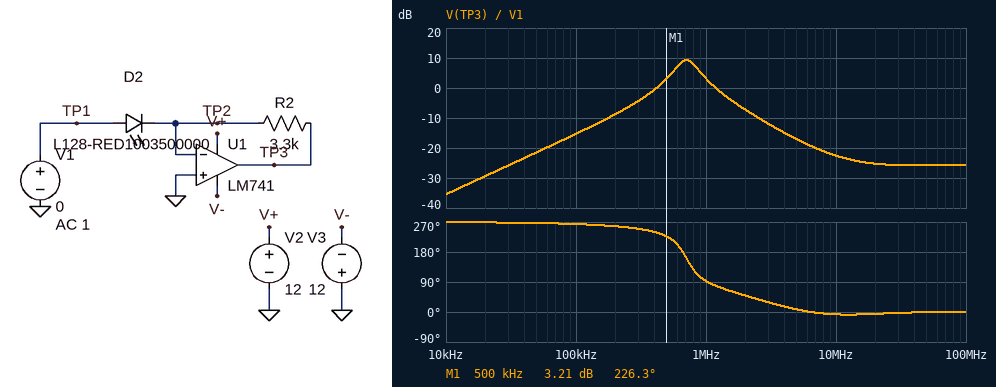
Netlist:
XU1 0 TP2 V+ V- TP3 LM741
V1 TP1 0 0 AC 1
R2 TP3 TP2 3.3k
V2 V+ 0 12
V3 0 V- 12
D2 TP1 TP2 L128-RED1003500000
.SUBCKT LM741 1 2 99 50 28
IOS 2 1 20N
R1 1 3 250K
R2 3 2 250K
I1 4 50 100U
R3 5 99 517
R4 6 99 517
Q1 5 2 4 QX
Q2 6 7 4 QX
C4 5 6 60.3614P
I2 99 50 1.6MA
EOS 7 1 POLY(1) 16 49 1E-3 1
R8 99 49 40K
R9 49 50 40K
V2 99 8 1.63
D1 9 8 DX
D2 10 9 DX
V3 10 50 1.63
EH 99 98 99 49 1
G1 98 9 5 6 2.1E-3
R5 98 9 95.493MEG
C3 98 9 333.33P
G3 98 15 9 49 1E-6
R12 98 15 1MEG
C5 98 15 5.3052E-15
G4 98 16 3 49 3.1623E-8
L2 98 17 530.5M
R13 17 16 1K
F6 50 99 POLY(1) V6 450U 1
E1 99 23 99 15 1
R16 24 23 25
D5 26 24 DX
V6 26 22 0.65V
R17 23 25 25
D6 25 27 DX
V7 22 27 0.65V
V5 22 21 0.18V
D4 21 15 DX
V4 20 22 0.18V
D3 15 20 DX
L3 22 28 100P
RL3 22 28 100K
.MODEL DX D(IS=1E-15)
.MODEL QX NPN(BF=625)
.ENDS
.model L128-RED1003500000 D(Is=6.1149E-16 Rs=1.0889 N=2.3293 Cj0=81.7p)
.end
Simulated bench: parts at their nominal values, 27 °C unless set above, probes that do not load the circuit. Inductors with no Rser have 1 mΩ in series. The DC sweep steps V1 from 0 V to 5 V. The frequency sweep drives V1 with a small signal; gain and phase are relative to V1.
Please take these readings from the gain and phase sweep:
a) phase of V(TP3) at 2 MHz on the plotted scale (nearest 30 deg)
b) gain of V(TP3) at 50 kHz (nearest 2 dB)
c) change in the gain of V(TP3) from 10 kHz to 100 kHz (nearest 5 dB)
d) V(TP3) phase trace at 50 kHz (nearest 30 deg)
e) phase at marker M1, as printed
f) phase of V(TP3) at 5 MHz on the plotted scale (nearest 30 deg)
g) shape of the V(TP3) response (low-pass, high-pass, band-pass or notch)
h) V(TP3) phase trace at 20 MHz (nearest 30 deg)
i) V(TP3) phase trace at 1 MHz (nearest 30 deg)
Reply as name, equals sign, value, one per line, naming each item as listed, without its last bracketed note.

phase of V(TP3) at 2 MHz on the plotted scale = 60 deg
gain of V(TP3) at 50 kHz = -22 dB
change in the gain of V(TP3) from 10 kHz to 100 kHz = 20 dB
V(TP3) phase trace at 50 kHz = 270 deg
phase at marker M1, as printed = 226.3 deg
phase of V(TP3) at 5 MHz on the plotted scale = 0 deg
shape of the V(TP3) response = band-pass
V(TP3) phase trace at 20 MHz = 0 deg
V(TP3) phase trace at 1 MHz = 90 deg
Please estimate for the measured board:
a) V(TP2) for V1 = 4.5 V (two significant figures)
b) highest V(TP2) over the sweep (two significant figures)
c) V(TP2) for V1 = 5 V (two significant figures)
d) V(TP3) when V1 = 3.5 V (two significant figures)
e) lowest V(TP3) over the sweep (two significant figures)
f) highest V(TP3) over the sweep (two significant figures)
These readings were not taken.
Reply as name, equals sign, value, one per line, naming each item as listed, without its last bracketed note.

V(TP2) for V1 = 4.5 V = 2.7 V
highest V(TP2) over the sweep = 3.2 V
V(TP2) for V1 = 5 V = 3.2 V
V(TP3) when V1 = 3.5 V = -11 V
lowest V(TP3) over the sweep = -11 V
highest V(TP3) over the sweep = 1.3 mV
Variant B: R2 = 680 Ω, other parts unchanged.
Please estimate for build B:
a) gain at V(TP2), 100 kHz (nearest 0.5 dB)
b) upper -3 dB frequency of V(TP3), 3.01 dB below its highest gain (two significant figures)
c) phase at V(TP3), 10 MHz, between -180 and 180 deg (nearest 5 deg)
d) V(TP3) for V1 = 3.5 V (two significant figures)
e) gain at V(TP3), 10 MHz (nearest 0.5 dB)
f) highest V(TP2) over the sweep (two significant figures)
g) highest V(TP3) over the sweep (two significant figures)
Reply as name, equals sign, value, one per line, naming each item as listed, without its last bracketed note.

gain at V(TP2), 100 kHz = -47.0 dB
upper -3 dB frequency of V(TP3), 3.01 dB below its highest gain = 2.1 MHz
phase at V(TP3), 10 MHz, between -180 and 180 deg = 10 deg
V(TP3) for V1 = 3.5 V = -10 V
gain at V(TP3), 10 MHz = -13.0 dB
highest V(TP2) over the sweep = 3.1 V
highest V(TP3) over the sweep = 1.1 mV
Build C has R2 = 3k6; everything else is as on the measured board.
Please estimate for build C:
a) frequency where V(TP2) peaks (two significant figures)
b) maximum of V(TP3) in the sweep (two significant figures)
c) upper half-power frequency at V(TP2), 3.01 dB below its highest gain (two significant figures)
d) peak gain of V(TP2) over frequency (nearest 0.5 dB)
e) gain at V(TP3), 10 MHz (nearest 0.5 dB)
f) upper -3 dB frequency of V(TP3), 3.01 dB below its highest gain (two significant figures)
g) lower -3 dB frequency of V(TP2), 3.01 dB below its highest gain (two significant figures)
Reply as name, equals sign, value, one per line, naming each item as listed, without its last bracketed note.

frequency where V(TP2) peaks = 710 kHz
maximum of V(TP3) in the sweep = 1.4 mV
upper half-power frequency at V(TP2), 3.01 dB below its highest gain = 930 kHz
peak gain of V(TP2) over frequency = 7.5 dB
gain at V(TP3), 10 MHz = -23.0 dB
upper -3 dB frequency of V(TP3), 3.01 dB below its highest gain = 830 kHz
lower -3 dB frequency of V(TP2), 3.01 dB below its highest gain = 600 kHz
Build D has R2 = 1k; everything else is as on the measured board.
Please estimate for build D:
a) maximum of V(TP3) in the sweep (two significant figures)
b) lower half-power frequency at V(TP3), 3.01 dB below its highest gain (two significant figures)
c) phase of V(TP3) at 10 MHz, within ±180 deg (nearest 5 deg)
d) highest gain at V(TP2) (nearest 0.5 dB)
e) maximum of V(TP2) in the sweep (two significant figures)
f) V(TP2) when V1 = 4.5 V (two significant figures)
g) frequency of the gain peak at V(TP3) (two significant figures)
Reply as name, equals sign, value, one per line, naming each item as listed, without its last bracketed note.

maximum of V(TP3) in the sweep = 1.1 mV
lower half-power frequency at V(TP3), 3.01 dB below its highest gain = 800 kHz
phase of V(TP3) at 10 MHz, within ±180 deg = 5 deg
highest gain at V(TP2) = 1.5 dB
maximum of V(TP2) in the sweep = 3.1 V
V(TP2) when V1 = 4.5 V = 2.6 V
frequency of the gain peak at V(TP3) = 1.1 MHz
